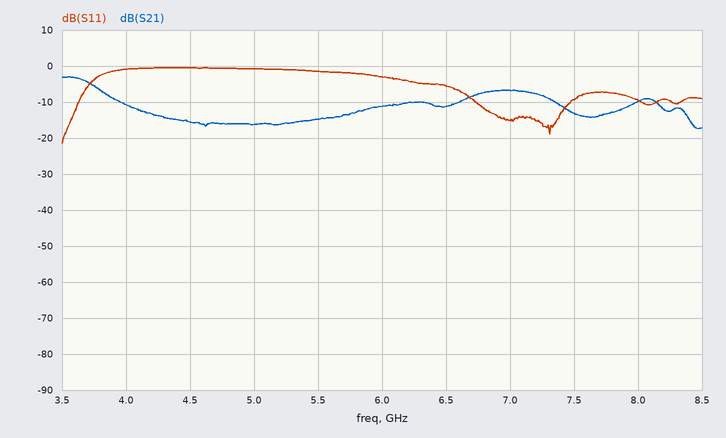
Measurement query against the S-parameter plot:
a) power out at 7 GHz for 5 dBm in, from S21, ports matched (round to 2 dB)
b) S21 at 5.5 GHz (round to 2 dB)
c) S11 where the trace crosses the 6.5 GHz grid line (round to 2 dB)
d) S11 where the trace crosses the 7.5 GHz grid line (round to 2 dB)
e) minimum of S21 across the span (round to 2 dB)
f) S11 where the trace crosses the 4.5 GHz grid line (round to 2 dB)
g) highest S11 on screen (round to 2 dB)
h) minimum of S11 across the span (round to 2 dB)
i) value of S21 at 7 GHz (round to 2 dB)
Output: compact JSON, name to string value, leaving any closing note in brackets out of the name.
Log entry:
{"power out at 7 GHz for 5 dBm in, from S21, ports matched": "-2 dBm", "S21 at 5.5 GHz": "-14 dB", "S11 where the trace crosses the 6.5 GHz grid line": "-6 dB", "S11 where the trace crosses the 7.5 GHz grid line": "-10 dB", "minimum of S21 across the span": "-18 dB", "S11 where the trace crosses the 4.5 GHz grid line": "0 dB", "highest S11 on screen": "0 dB", "minimum of S11 across the span": "-22 dB", "value of S21 at 7 GHz": "-6 dB"}
